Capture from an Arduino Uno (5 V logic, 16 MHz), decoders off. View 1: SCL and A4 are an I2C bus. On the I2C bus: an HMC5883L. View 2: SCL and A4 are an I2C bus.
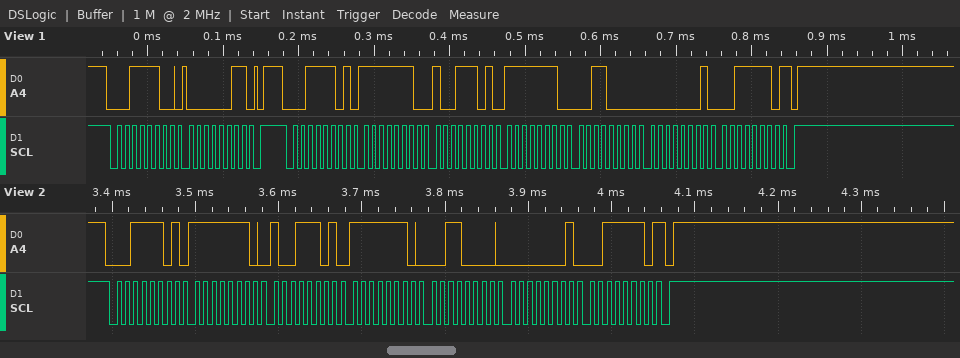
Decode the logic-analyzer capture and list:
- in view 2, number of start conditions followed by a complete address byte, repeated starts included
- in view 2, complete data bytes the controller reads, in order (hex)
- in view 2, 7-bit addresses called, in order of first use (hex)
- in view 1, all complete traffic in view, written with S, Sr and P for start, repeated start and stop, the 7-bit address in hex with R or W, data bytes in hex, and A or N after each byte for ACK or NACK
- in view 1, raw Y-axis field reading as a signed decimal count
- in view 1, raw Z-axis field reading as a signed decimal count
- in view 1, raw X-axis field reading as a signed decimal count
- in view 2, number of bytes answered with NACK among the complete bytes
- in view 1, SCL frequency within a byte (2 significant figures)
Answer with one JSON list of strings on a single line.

["1", "FE 9D FE 30 01 3E", "0x1E", "S 1EW A 03 A P S 1ER A FE A 9D A FE A 30 A 01 A 3E N P", "318", "-464", "-355", "1", "100 kHz"]
